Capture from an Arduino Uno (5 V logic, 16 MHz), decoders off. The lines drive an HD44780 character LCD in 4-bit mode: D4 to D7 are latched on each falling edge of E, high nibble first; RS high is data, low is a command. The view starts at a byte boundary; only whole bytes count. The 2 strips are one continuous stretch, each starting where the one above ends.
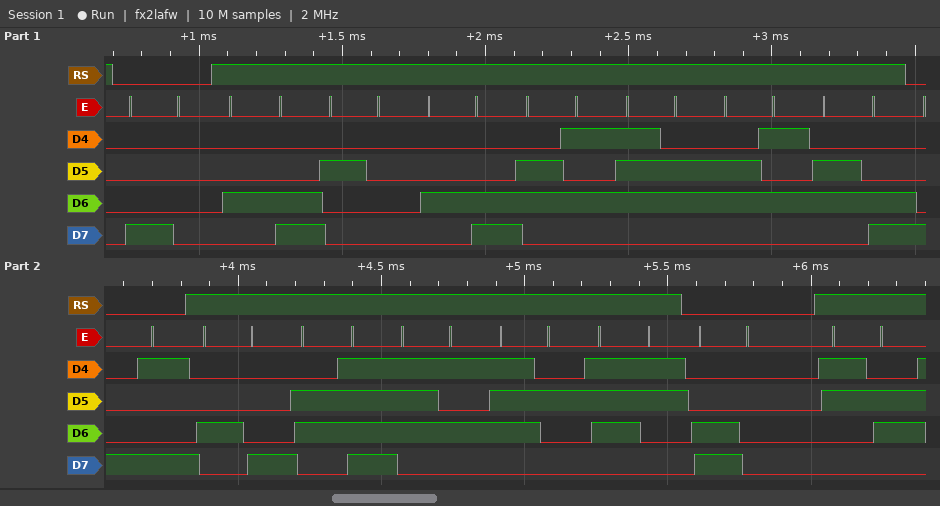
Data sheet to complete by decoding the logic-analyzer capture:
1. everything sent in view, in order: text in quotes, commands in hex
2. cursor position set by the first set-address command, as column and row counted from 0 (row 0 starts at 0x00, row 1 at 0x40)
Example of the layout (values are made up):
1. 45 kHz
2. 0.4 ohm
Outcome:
1. 0x80 "L Level" 0x89 "Hours" 0xC0 "6"
2. column 0, row 0
